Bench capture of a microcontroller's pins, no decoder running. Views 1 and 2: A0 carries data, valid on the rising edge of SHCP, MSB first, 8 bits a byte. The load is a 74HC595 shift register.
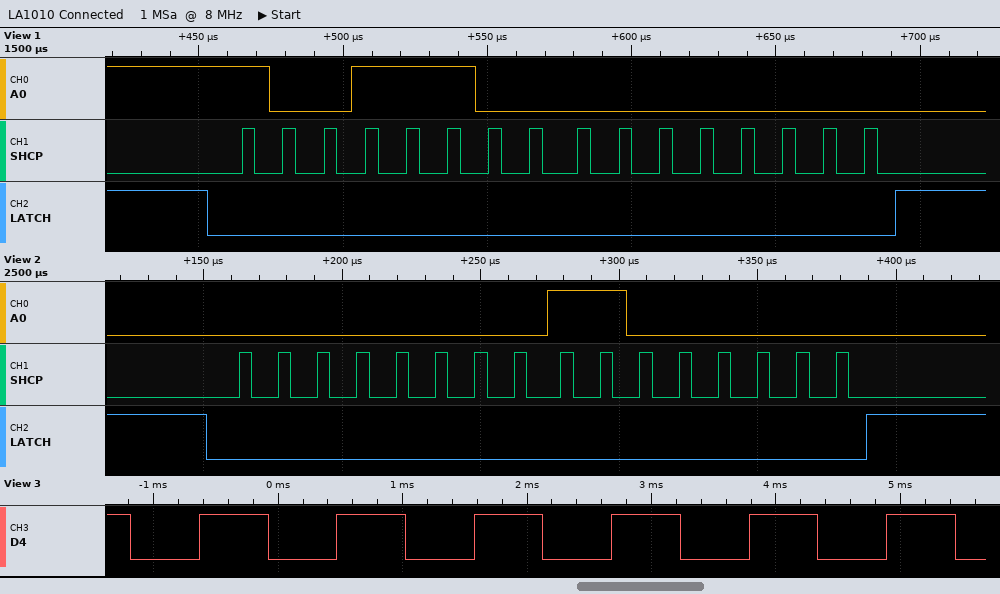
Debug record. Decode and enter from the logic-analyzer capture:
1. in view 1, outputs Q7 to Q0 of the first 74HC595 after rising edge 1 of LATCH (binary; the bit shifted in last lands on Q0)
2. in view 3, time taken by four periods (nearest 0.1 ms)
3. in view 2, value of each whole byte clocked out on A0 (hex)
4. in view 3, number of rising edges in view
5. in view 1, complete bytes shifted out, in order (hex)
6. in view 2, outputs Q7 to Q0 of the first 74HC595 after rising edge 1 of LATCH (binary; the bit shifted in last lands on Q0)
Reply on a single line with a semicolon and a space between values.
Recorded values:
00000000; 4.4 ms; 0x00 0xC0; 6; 9C 00; 11000000
